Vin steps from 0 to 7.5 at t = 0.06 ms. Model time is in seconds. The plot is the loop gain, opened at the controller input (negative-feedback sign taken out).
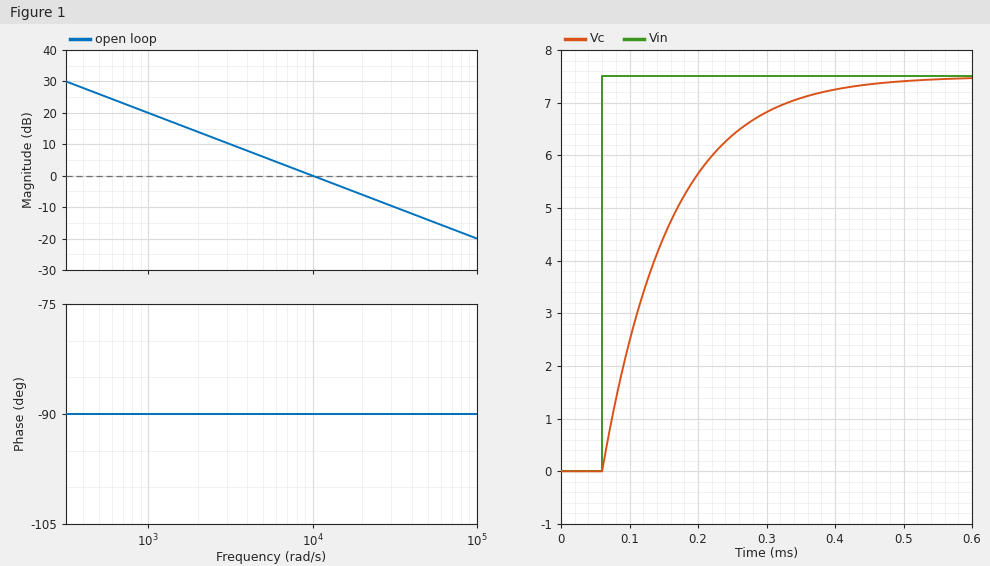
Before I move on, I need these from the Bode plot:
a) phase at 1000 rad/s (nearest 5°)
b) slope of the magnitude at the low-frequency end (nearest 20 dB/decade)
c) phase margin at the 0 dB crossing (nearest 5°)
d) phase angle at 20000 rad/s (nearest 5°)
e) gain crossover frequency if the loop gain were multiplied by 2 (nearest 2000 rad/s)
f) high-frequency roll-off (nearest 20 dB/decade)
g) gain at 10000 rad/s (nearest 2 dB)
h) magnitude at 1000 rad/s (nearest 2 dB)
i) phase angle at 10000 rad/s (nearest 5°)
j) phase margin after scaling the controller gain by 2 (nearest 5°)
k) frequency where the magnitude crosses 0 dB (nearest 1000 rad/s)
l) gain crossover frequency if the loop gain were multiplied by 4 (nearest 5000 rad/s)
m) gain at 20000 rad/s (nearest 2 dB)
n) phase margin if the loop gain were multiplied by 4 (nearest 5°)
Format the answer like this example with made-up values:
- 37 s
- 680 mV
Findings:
- -90°
- -20 dB/decade
- 90°
- -90°
- 20000 rad/s
- -20 dB/decade
- 0 dB
- 20 dB
- -90°
- 90°
- 10000 rad/s
- 40000 rad/s
- -6 dB
- 90°
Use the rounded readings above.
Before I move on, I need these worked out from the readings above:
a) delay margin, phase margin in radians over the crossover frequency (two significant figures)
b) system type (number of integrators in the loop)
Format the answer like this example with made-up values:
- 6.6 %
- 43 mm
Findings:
- 0.00016 s
- 1
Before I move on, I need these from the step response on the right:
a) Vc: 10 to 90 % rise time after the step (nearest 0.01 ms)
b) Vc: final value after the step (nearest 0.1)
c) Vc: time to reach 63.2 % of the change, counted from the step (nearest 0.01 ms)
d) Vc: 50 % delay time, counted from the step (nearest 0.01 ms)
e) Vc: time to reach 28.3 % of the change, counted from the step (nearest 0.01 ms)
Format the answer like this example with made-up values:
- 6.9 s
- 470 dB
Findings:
- 0.22 ms
- 7.5
- 0.10 ms
- 0.07 ms
- 0.03 ms
